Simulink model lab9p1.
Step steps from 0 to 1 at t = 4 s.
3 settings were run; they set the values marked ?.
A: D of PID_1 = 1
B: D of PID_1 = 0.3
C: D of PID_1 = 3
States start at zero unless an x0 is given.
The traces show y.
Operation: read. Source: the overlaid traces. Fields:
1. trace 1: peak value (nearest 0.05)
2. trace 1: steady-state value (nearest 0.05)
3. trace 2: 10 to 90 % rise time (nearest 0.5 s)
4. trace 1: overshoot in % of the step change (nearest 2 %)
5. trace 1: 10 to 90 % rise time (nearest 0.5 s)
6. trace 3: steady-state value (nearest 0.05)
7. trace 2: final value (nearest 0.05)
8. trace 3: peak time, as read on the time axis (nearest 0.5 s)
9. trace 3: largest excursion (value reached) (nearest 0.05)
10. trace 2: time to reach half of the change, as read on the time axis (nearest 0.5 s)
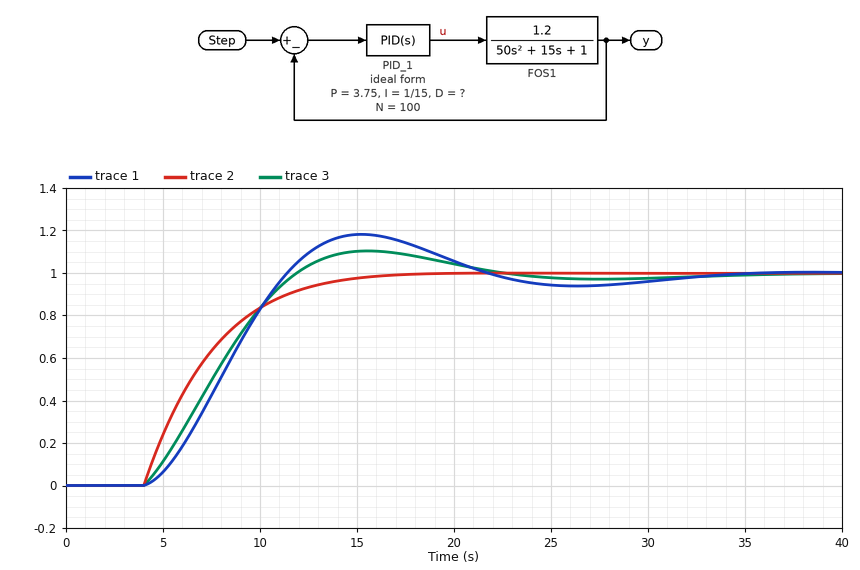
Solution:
1.20
1.00
7.0 s
18 %
5.0 s
1.00
1.00
15.5 s
1.10
6.5 s
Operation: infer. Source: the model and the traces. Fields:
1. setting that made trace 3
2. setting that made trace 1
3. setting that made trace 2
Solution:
A
B
C
